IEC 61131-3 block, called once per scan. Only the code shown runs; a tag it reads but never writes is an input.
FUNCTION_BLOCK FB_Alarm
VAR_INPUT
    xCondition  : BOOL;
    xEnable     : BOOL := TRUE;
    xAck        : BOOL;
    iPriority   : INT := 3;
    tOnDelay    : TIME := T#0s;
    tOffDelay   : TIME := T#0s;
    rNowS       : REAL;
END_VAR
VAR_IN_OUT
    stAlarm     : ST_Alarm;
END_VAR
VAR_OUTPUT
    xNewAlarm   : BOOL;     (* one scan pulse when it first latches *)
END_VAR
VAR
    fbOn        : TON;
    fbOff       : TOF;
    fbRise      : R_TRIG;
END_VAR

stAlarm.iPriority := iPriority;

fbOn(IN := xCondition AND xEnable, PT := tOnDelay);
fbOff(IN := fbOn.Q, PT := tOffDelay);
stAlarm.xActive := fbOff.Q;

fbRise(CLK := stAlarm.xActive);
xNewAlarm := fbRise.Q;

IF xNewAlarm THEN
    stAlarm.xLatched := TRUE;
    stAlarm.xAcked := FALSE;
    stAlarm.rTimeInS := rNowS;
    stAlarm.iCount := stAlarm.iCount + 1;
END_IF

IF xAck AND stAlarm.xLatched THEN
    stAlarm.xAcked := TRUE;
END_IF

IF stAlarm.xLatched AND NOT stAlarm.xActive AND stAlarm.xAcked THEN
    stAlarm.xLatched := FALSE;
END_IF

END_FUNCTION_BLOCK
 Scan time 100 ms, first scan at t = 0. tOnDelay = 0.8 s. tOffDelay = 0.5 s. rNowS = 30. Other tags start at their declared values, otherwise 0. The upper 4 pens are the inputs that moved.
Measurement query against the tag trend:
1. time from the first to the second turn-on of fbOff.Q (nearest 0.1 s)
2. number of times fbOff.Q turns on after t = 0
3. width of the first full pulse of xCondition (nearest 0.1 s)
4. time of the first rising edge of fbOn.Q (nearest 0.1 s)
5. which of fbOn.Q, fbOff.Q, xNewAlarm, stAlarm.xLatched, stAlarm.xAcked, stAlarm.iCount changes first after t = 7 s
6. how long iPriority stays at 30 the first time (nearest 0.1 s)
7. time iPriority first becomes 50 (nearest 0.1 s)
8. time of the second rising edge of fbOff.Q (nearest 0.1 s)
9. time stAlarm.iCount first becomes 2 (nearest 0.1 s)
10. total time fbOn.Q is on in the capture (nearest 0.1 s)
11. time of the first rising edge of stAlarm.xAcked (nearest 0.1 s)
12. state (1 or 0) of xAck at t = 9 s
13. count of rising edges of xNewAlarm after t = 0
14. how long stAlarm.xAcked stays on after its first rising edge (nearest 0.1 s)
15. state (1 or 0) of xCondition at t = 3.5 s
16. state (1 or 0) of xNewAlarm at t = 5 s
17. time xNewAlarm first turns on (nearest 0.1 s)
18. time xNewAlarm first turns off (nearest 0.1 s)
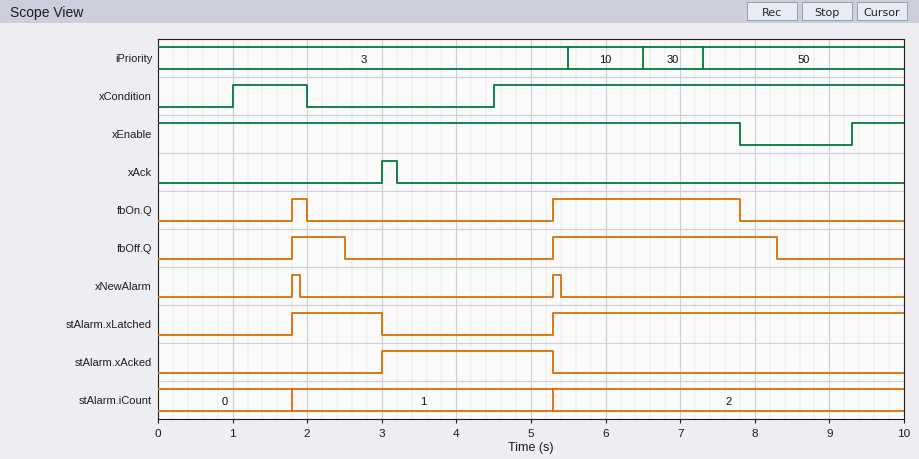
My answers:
3.5 s
2
1.0 s
1.8 s
fbOn.Q
0.8 s
7.3 s
5.3 s
5.3 s
2.7 s
3.0 s
0
2
2.3 s
0
0
1.8 s
1.9 s
